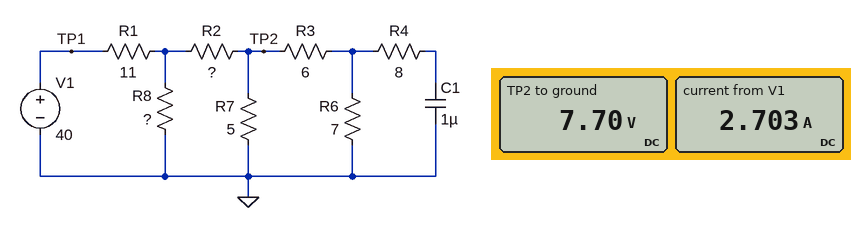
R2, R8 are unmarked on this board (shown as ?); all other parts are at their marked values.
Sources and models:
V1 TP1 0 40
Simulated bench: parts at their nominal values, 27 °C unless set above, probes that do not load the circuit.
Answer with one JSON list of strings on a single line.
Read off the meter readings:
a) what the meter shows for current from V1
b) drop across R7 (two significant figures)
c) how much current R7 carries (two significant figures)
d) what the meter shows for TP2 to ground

["2.703 A", "7.7 V", "1.5 A", "7.70 V"]
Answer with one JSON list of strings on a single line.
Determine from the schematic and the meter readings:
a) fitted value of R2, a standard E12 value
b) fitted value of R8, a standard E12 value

["1.2 Ω", "18 Ω"]
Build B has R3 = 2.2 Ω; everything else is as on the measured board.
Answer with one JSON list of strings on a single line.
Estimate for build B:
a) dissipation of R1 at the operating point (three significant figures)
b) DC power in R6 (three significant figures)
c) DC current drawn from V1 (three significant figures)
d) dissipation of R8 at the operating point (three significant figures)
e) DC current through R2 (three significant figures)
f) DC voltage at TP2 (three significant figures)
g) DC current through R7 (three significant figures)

["83.0 W", "4.21 W", "2.75 A", "5.32 W", "2.20 A", "7.14 V", "1.43 A"]
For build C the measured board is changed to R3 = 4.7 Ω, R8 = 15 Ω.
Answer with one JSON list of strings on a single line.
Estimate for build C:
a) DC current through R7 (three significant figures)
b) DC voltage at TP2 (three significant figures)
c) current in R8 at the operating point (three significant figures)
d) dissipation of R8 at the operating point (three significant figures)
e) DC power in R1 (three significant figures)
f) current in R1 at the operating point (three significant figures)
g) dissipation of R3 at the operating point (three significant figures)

["1.46 A", "7.32 V", "655 mA", "6.43 W", "82.8 W", "2.74 A", "1.84 W"]
